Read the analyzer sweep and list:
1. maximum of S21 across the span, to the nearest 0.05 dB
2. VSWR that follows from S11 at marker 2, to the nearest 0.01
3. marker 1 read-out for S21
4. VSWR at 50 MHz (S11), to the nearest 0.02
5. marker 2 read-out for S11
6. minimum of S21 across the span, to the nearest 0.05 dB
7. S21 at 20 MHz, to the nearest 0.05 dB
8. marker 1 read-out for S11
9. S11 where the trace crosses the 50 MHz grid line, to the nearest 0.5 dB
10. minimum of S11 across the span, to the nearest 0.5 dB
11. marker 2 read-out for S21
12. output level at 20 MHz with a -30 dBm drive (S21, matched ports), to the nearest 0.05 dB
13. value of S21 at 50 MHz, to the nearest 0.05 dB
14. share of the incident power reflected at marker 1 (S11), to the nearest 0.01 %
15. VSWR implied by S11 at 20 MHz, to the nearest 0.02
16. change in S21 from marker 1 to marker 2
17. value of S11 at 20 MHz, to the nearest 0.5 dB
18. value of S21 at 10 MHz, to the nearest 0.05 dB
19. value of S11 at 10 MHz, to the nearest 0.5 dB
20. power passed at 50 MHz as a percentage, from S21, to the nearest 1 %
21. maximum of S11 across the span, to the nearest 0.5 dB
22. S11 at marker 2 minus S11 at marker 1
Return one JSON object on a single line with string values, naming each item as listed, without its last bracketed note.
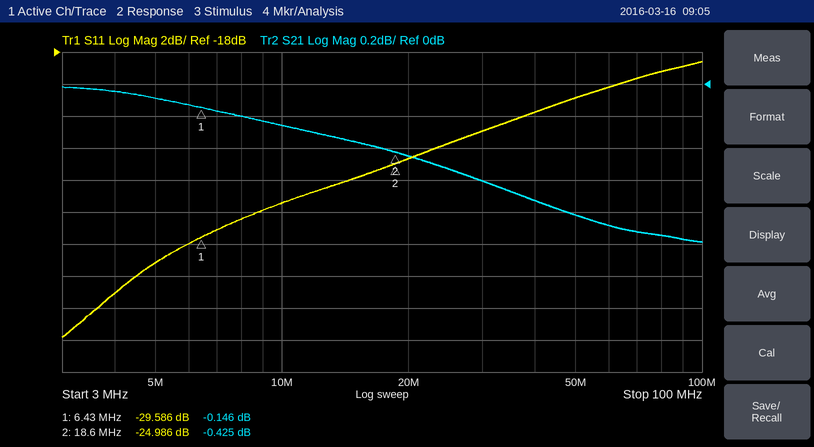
{"maximum of S21 across the span, to the nearest 0.05 dB": "0.00 dB", "VSWR that follows from S11 at marker 2, to the nearest 0.01": "1.12", "marker 1 read-out for S21": "-0.146 dB", "VSWR at 50 MHz (S11), to the nearest 0.02": "1.20", "marker 2 read-out for S11": "-24.986 dB", "minimum of S21 across the span, to the nearest 0.05 dB": "-1.00 dB", "S21 at 20 MHz, to the nearest 0.05 dB": "-0.45 dB", "marker 1 read-out for S11": "-29.586 dB", "S11 where the trace crosses the 50 MHz grid line, to the nearest 0.5 dB": "-21.0 dB", "minimum of S11 across the span, to the nearest 0.5 dB": "-36.0 dB", "marker 2 read-out for S21": "-0.425 dB", "output level at 20 MHz with a -30 dBm drive (S21, matched ports), to the nearest 0.05 dB": "-30.45 dBm", "value of S21 at 50 MHz, to the nearest 0.05 dB": "-0.80 dB", "share of the incident power reflected at marker 1 (S11), to the nearest 0.01 %": "0.11 %", "VSWR implied by S11 at 20 MHz, to the nearest 0.02": "1.12", "change in S21 from marker 1 to marker 2": "-0.279 dB", "value of S11 at 20 MHz, to the nearest 0.5 dB": "-24.5 dB", "value of S21 at 10 MHz, to the nearest 0.05 dB": "-0.25 dB", "value of S11 at 10 MHz, to the nearest 0.5 dB": "-27.5 dB", "power passed at 50 MHz as a percentage, from S21, to the nearest 1 %": "83 %", "maximum of S11 across the span, to the nearest 0.5 dB": "-18.5 dB", "S11 at marker 2 minus S11 at marker 1": "4.600 dB"}
